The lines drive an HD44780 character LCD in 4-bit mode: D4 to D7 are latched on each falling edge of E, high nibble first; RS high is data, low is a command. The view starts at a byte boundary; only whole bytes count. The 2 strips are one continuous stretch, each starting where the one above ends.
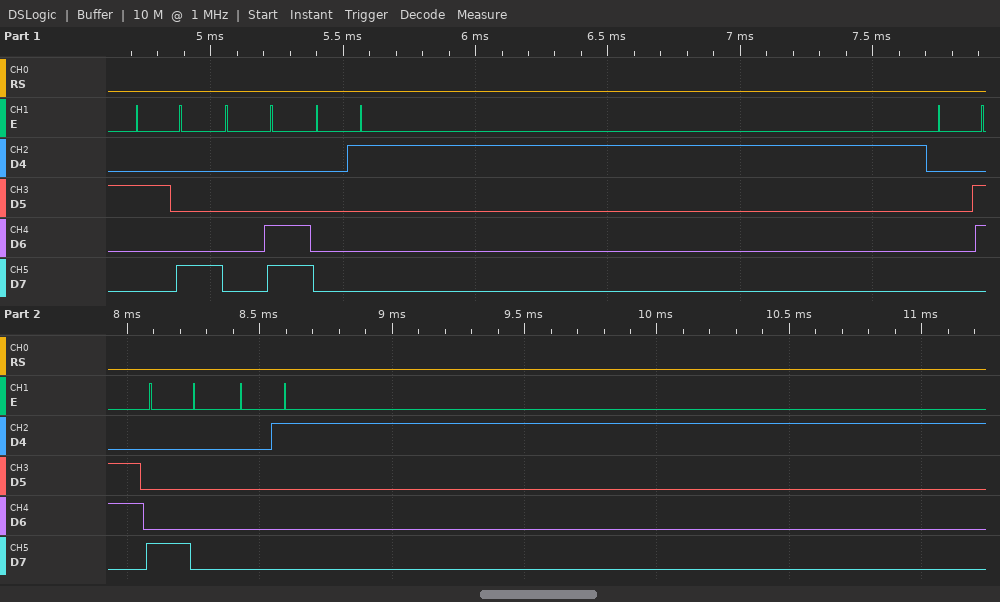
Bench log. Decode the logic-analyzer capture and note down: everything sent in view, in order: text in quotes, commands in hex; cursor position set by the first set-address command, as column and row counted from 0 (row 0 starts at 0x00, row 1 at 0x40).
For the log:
0x28 0x0C 0x01 0x06 0x80 0x01
column 0, row 0
